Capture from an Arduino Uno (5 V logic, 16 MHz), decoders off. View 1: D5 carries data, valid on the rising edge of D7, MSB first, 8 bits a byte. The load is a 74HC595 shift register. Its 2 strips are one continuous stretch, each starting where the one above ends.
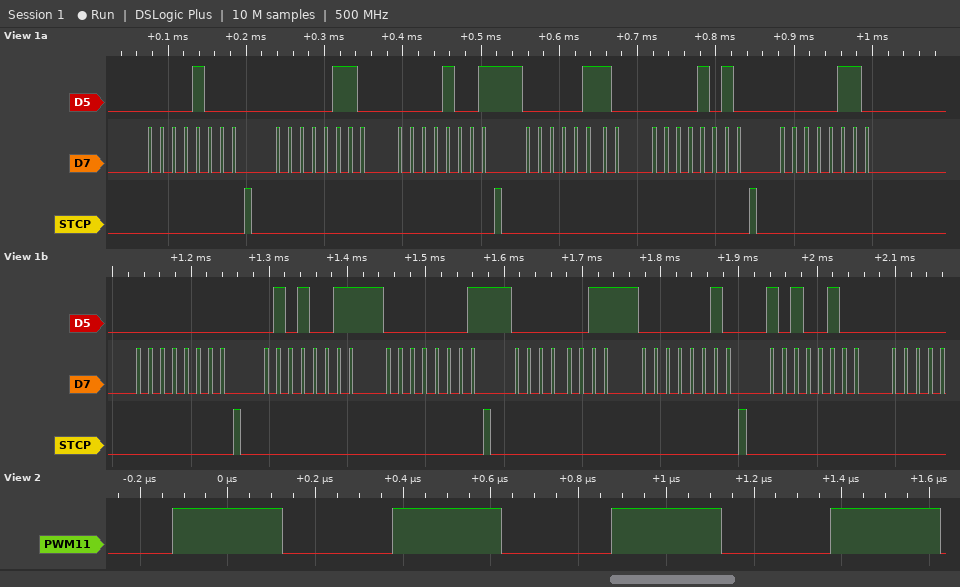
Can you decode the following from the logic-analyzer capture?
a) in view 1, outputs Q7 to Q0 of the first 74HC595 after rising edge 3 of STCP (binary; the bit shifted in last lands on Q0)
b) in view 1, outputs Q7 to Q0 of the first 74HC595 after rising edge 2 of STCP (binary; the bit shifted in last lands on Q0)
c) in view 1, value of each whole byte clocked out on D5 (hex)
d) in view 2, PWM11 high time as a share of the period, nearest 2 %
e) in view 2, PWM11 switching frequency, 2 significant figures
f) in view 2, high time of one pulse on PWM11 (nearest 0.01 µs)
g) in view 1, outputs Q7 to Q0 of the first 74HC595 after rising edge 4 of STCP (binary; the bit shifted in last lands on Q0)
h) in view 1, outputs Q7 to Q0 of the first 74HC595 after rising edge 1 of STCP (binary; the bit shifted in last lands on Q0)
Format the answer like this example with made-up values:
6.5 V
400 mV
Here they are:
00001010
00001001
08 06 09 06 0A 06 00 53 01 03 02 A4
50 %
2.0 MHz
0.25 µs
00000000
00001000
